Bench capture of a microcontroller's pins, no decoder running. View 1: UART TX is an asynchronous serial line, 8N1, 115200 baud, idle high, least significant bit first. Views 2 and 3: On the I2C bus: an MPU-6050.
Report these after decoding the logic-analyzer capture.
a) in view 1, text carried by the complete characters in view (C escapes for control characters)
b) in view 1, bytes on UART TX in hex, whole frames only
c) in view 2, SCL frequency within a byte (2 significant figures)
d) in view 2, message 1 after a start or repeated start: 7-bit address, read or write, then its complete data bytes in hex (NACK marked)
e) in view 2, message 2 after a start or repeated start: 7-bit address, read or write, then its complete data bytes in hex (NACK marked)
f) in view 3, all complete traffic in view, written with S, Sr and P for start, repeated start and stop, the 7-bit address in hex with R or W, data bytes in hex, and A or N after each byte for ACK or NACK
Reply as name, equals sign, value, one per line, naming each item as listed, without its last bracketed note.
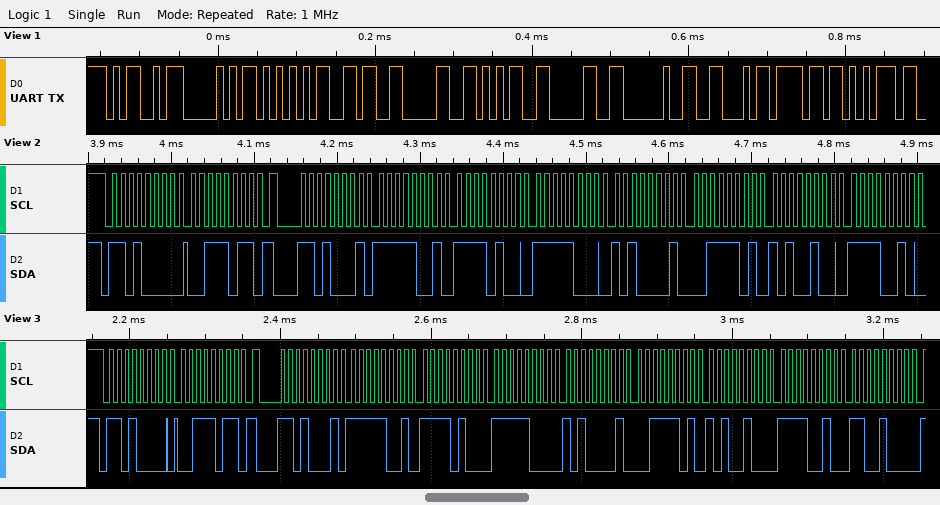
in view 1, text carried by the complete characters in view = "MPU6050 Fou"
in view 1, bytes on UART TX in hex, whole frames only = 4D 50 55 36 30 35 30 20 46 6F 75
in view 2, SCL frequency within a byte = 100 kHz
in view 2, message 1 after a start or repeated start: 7-bit address, read or write, then its complete data bytes in hex = 0x68 write: 3B
in view 2, message 2 after a start or repeated start: 7-bit address, read or write, then its complete data bytes in hex = 0x68 read: F9 F4 F8 A1 3D A4 F2
in view 3, all complete traffic in view, written with S, Sr and P for start, repeated start and stop, the 7-bit address in hex with R or W, data bytes in hex, and A or N after each byte for ACK or NACK = S 68W A 3B A Sr 68R A F9 A F4 A F8 A A1 A 3D A A4 A F2 A C8 A
